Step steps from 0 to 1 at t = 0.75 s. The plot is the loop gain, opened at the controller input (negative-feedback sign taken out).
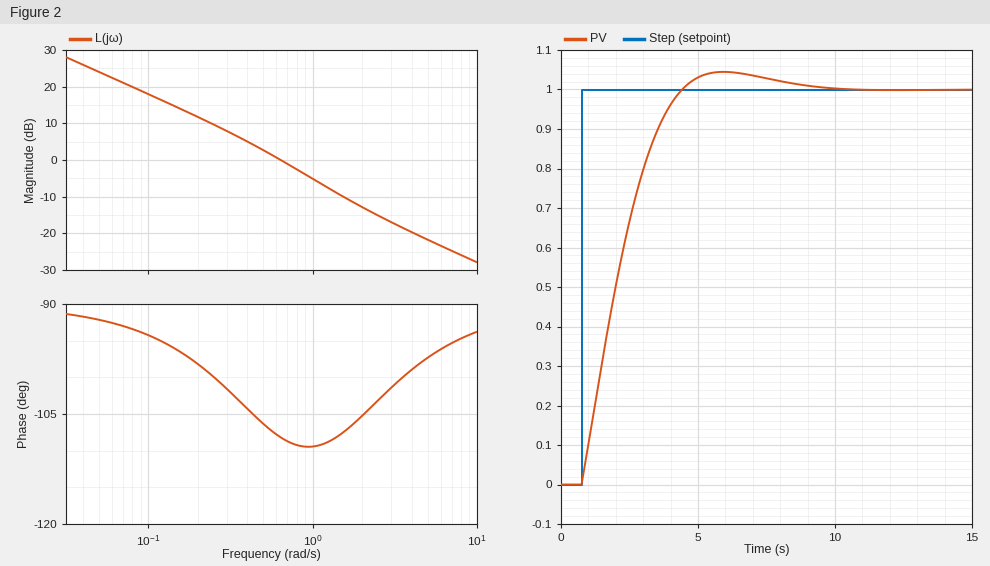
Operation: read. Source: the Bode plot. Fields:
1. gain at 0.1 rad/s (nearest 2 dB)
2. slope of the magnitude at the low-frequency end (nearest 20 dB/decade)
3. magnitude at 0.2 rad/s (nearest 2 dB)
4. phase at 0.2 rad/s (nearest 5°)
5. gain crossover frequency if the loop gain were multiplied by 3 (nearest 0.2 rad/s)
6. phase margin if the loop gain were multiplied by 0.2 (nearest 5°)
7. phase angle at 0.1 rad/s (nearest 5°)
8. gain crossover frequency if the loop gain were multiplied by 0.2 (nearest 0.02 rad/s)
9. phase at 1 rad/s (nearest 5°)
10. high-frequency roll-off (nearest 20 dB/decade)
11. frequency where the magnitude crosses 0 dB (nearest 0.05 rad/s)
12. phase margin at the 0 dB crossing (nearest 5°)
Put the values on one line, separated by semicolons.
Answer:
18 dB; -20 dB/decade; 12 dB; -100°; 1.4 rad/s; 85°; -95°; 0.16 rad/s; -110°; -20 dB/decade; 0.65 rad/s; 70°
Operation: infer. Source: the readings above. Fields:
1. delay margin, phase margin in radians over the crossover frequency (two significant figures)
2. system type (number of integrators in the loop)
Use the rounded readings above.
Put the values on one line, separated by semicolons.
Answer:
1.9 s; 1
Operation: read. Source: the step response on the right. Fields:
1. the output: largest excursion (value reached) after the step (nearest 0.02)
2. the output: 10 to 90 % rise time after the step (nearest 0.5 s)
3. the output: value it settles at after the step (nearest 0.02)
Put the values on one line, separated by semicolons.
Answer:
1.04; 2.5 s; 1.00
